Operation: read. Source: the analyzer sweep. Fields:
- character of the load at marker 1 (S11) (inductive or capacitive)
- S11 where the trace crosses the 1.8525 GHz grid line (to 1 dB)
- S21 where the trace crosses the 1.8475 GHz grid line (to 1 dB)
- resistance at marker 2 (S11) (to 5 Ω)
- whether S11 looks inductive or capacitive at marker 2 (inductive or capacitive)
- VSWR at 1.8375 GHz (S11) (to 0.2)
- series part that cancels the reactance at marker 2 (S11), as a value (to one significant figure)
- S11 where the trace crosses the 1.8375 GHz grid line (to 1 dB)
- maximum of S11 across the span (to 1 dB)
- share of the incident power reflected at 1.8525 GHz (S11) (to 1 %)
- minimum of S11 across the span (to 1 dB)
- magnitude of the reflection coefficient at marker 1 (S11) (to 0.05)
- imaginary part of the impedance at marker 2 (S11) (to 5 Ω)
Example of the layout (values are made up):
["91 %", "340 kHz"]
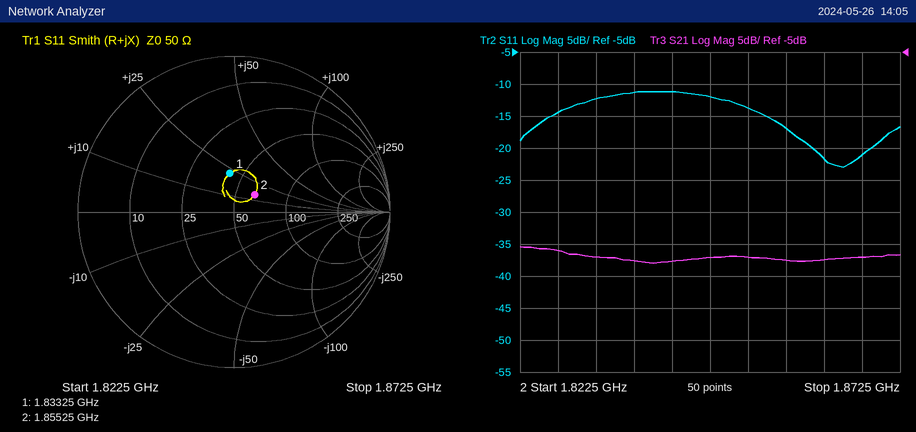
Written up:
["inductive", "-14 dB", "-37 dB", "65 Ω", "inductive", "1.8", "6 pF", "-11 dB", "-11 dB", "4 %", "-23 dB", "0.25", "+15 Ω"]
